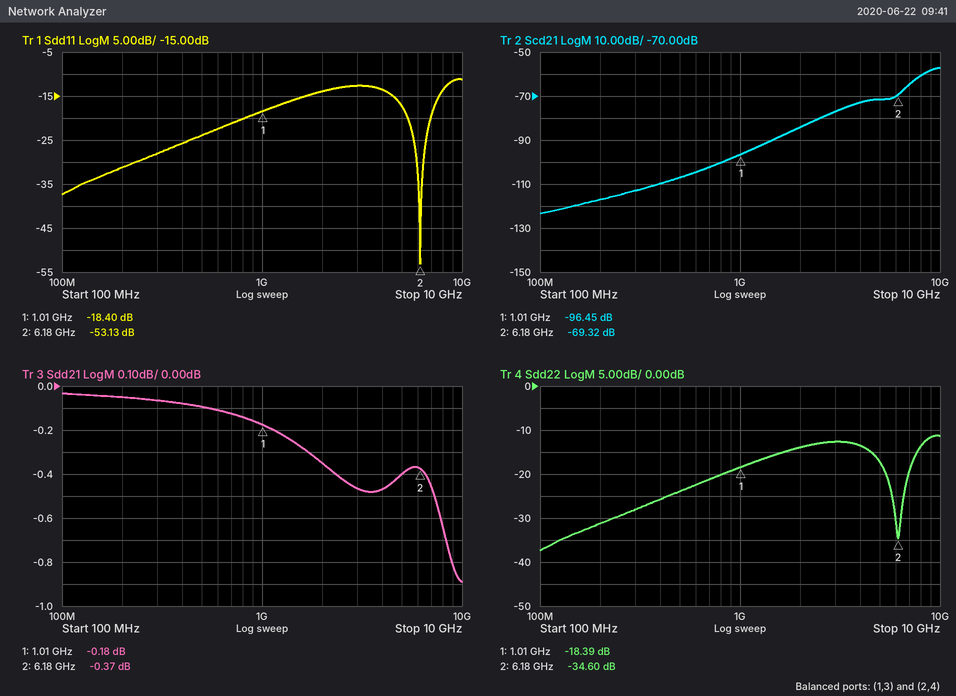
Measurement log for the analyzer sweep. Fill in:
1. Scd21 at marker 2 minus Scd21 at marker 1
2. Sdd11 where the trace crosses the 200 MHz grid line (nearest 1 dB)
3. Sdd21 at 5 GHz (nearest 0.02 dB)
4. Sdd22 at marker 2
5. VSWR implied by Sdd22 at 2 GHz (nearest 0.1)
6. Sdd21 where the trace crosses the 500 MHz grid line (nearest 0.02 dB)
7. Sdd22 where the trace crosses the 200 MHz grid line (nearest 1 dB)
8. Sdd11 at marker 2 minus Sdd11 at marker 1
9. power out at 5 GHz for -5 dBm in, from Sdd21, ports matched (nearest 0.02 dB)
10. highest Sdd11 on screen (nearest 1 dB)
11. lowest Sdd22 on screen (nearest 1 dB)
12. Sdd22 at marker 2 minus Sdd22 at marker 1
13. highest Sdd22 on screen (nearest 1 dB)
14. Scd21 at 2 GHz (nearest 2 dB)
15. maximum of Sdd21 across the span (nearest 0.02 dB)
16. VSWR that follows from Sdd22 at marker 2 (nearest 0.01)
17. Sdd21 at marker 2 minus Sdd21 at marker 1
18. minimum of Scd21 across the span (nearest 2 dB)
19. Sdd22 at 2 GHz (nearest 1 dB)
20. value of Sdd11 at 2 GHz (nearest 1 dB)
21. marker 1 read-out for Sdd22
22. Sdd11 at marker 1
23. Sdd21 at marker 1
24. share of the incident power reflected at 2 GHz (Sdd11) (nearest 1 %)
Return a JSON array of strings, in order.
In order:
["27.13 dB", "-31 dB", "-0.40 dB", "-34.60 dB", "1.5", "-0.10 dB", "-31 dB", "-34.73 dB", "-5.40 dBm", "-11 dB", "-37 dB", "-16.21 dB", "-11 dB", "-84 dB", "-0.04 dB", "1.04", "-0.19 dB", "-124 dB", "-14 dB", "-14 dB", "-18.39 dB", "-18.40 dB", "-0.18 dB", "4 %"]
